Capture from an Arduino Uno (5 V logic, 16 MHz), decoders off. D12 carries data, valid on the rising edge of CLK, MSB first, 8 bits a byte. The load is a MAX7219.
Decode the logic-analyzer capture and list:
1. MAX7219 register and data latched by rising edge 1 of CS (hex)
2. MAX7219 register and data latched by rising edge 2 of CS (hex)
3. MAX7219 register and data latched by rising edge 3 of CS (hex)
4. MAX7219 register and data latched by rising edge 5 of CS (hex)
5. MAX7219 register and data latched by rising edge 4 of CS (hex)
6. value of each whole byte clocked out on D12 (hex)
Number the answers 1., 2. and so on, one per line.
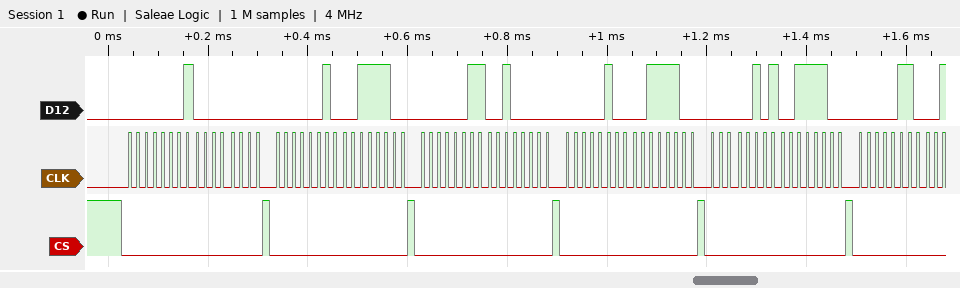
1. register 0x1, data 0x00
2. register 0x2, data 0x3C
3. register 0x3, data 0x20
4. register 0x5, data 0x3C
5. register 0x4, data 0x3C
6. 0x01 0x00 0x02 0x3C 0x03 0x20 0x04 0x3C 0x05 0x3C 0x06
